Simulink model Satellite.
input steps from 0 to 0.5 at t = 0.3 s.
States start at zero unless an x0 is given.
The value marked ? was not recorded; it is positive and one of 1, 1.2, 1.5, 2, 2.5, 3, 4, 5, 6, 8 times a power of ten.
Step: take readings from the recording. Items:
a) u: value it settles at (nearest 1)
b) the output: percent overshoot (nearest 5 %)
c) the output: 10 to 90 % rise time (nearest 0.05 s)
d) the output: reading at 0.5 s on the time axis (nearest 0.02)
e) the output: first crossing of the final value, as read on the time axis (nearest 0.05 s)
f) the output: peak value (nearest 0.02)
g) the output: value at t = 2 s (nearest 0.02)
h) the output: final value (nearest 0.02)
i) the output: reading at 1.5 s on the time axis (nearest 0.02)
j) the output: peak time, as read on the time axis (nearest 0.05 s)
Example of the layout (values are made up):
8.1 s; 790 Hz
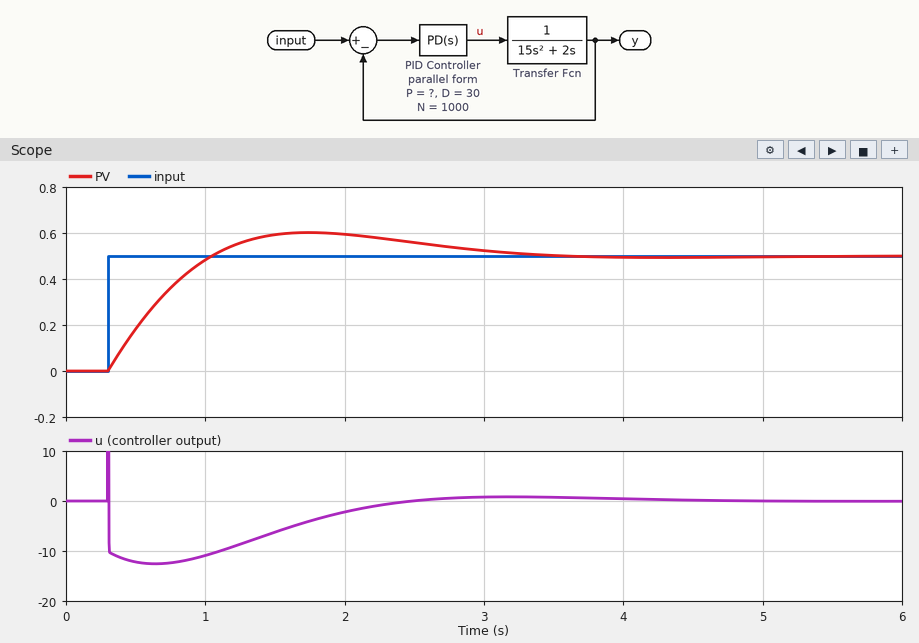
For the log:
0; 20 %; 0.55 s; 0.18; 1.05 s; 0.60; 0.60; 0.50; 0.60; 1.75 s
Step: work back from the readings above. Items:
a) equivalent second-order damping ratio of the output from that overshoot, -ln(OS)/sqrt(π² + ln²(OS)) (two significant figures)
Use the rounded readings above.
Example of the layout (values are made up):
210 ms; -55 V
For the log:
0.46
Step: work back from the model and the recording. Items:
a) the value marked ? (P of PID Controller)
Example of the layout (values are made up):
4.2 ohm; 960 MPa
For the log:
40
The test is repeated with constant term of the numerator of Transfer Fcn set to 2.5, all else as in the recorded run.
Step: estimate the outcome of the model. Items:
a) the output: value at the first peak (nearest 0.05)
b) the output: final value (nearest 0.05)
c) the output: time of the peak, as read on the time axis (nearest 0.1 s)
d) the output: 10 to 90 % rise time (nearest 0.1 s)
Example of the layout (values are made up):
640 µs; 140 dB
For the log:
0.55; 0.50; 1.1 s; 0.3 s
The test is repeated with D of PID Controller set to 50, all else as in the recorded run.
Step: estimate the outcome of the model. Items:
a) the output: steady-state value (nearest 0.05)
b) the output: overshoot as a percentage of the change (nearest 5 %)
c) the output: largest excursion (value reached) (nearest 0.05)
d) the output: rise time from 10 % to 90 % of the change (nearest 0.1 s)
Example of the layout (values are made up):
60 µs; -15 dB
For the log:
0.50; 10 %; 0.55; 0.5 s
